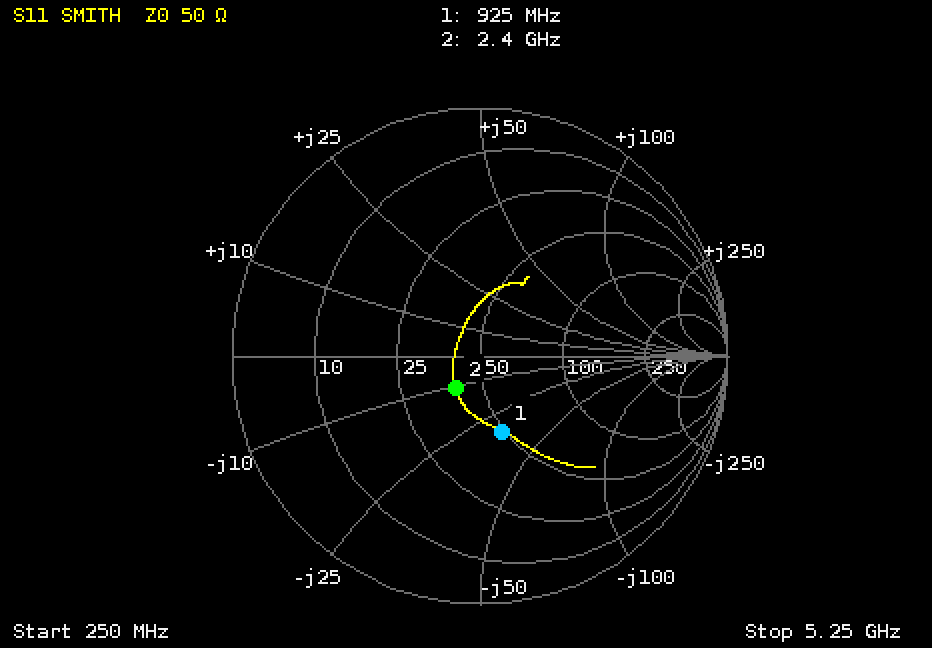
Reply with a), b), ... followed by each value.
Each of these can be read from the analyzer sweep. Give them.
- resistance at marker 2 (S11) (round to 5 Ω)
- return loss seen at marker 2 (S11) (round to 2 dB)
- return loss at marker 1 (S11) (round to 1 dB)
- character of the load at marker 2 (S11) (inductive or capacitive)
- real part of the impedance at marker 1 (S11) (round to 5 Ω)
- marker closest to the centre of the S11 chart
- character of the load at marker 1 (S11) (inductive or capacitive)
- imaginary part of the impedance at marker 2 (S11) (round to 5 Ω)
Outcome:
a) 40 Ω
b) 16 dB
c) 10 dB
d) capacitive
e) 50 Ω
f) marker 2
g) capacitive
h) -10 Ω
